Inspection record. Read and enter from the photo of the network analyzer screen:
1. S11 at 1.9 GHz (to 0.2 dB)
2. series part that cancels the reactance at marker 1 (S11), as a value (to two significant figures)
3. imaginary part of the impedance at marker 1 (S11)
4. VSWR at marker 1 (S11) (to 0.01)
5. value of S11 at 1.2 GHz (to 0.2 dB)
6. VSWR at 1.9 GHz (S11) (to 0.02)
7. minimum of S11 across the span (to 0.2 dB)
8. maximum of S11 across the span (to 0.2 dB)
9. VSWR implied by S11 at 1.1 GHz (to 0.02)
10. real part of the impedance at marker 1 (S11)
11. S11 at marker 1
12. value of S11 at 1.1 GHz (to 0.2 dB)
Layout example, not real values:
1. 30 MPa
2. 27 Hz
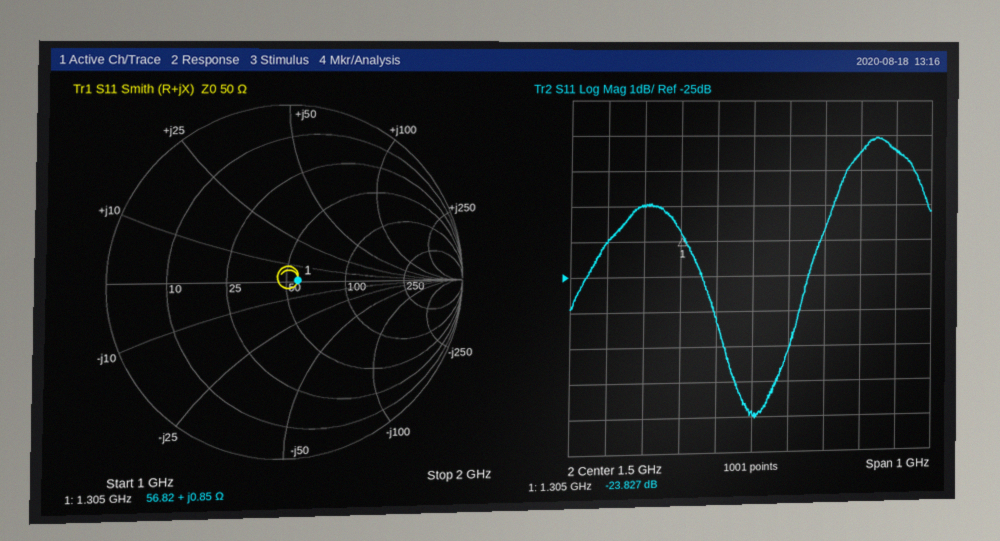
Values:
1. -21.4 dB
2. 140 pF
3. +0.85 Ω
4. 1.14
5. -23.0 dB
6. 1.18
7. -29.0 dB
8. -21.0 dB
9. 1.14
10. 56.82 Ω
11. -23.827 dB
12. -24.0 dB
